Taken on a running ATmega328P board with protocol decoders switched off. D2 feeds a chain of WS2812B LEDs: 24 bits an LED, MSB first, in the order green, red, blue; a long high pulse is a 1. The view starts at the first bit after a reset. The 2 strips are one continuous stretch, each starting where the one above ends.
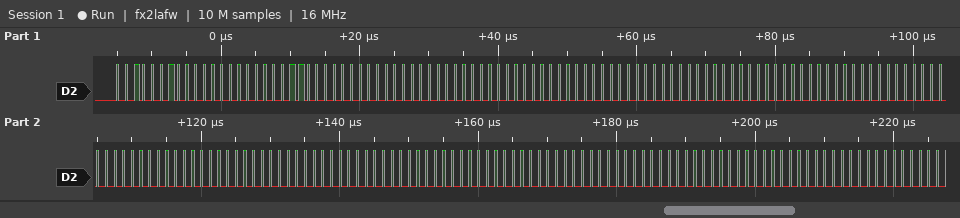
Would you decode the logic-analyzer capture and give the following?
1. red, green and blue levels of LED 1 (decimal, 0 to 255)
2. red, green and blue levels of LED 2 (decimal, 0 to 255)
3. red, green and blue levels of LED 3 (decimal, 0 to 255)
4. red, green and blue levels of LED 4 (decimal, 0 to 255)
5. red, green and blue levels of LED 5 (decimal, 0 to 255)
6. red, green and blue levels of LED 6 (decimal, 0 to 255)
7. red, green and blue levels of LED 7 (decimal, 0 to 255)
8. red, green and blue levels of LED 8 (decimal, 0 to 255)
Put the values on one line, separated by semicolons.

0, 34, 12; 0, 0, 0; 0, 0, 0; 0, 0, 0; 0, 0, 0; 0, 0, 0; 0, 0, 0; 0, 0, 0
